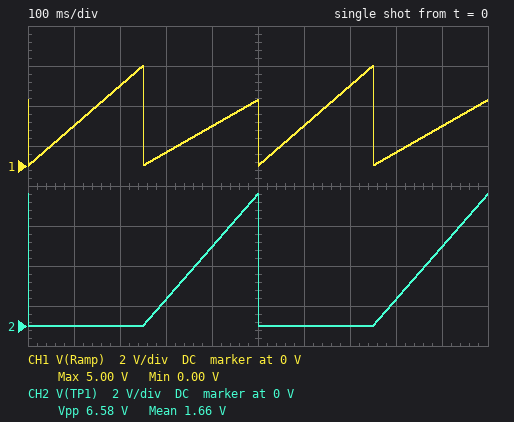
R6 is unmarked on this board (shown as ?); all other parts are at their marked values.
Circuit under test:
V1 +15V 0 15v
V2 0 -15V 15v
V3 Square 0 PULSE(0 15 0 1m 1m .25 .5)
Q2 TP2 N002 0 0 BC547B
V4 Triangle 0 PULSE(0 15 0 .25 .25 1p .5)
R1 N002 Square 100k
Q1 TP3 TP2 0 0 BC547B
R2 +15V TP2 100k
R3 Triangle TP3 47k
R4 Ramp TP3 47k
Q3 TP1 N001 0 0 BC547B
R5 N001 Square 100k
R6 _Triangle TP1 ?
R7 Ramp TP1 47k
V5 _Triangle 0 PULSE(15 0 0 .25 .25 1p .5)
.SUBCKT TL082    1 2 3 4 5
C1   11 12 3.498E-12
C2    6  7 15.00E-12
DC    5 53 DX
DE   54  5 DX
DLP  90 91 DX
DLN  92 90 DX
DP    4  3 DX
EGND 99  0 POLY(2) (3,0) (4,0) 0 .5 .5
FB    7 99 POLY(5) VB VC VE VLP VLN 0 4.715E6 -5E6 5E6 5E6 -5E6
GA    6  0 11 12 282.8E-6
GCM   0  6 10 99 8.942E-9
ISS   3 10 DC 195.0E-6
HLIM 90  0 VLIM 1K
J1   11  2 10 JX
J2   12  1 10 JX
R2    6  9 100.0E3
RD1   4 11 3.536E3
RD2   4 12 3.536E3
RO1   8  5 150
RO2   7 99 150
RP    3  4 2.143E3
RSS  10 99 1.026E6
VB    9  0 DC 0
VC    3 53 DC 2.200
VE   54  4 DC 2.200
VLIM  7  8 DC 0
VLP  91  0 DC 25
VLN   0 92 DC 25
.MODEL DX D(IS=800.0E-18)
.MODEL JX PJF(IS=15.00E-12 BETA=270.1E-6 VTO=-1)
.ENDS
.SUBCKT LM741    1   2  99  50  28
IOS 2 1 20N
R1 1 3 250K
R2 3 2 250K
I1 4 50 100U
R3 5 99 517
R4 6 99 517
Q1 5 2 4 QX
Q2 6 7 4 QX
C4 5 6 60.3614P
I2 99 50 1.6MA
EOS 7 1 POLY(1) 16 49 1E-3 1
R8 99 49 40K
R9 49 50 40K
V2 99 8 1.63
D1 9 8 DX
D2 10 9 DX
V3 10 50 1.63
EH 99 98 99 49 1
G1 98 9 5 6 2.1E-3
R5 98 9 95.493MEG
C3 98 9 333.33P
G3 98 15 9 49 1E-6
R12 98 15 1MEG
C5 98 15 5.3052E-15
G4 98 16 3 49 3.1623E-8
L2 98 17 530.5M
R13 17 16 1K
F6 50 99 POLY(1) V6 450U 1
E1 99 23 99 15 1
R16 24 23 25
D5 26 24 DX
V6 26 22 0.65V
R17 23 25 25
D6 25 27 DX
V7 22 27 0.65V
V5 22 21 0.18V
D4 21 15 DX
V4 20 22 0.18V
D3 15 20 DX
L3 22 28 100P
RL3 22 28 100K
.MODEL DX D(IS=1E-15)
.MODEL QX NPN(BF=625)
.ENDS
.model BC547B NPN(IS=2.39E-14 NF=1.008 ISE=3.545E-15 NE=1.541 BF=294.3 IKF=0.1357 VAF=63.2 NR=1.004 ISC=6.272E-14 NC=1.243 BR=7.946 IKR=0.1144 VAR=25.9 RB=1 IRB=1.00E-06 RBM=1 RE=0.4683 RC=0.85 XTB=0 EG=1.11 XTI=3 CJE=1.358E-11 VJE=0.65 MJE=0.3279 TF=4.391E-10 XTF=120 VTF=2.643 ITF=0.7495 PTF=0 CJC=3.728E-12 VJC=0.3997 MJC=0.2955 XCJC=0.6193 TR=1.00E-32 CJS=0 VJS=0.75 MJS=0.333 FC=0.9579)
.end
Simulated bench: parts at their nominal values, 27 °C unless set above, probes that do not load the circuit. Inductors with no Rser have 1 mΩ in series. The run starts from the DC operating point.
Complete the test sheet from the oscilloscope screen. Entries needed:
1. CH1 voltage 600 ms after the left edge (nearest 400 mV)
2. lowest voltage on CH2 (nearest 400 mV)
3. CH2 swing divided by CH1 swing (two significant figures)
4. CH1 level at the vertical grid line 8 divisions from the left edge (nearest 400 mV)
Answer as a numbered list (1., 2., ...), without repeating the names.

1. 2.0 V
2. 0 V
3. 1.3
4. 800 mV
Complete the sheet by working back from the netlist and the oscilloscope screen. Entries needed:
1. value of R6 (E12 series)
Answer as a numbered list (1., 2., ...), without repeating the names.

1. 120 kΩ
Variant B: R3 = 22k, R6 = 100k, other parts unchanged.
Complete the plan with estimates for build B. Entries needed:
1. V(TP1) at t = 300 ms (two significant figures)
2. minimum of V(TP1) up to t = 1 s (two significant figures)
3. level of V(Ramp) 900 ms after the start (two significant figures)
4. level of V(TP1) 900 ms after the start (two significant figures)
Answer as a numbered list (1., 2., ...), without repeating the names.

1. 1.5 V
2. 9.7 mV
3. 2.2 V
4. 4.4 V
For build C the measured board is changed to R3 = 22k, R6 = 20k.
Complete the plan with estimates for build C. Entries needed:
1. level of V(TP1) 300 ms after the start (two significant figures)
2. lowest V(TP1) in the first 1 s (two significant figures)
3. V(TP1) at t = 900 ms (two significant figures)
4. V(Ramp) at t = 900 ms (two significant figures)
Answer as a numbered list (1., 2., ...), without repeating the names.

1. 2.5 V
2. 9.7 mV
3. 7.4 V
4. 3.7 V
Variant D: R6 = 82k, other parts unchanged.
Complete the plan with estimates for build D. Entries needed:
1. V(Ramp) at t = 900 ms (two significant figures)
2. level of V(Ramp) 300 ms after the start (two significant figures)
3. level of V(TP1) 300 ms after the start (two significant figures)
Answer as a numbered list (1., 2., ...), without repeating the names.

1. 2.4 V
2. 810 mV
3. 1.6 V
